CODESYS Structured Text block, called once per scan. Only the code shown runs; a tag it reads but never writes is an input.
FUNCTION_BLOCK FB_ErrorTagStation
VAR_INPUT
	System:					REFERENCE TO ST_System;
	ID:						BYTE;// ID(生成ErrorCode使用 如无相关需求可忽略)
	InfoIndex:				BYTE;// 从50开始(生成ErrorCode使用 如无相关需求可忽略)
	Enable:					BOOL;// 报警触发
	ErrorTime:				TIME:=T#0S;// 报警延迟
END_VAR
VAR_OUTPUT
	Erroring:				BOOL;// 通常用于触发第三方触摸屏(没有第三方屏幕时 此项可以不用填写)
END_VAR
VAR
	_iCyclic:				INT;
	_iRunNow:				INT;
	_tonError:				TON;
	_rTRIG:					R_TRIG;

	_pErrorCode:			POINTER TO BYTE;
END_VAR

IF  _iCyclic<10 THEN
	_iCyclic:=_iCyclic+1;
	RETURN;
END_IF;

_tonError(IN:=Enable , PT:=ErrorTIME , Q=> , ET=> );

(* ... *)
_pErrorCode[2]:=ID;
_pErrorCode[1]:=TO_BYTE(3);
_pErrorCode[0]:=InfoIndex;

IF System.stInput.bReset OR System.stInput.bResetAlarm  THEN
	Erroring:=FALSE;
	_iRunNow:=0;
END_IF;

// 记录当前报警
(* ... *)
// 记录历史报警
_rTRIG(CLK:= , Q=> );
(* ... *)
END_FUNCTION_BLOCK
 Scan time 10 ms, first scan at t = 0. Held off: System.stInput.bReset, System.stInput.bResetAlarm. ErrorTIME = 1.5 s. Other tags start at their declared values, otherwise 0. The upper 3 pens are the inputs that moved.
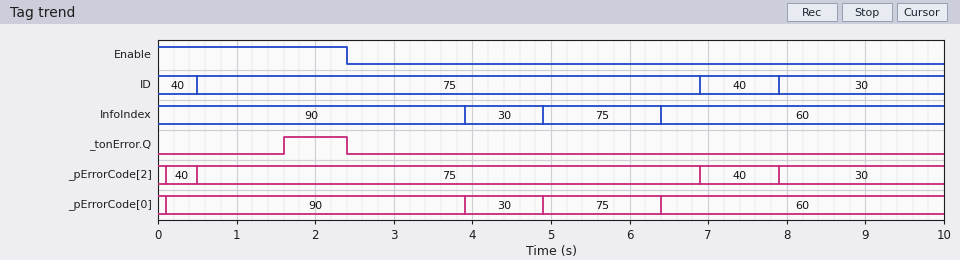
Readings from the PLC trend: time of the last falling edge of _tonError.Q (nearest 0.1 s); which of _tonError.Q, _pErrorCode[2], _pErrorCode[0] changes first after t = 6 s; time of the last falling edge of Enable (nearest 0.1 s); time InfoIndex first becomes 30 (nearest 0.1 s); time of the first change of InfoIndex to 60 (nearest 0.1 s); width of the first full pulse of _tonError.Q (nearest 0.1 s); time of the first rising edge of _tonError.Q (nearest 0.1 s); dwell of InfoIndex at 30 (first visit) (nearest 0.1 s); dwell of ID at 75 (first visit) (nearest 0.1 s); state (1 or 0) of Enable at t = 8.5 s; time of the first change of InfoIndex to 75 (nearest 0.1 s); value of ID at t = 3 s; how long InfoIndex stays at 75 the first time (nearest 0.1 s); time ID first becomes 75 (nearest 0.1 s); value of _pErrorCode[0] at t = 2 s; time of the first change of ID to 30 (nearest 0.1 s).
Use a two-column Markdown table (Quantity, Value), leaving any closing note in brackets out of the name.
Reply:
| Quantity | Value |
|---|---|
| time of the last falling edge of _tonError.Q | 2.4 s |
| which of _tonError.Q, _pErrorCode[2], _pErrorCode[0] changes first after t = 6 s | _pErrorCode[0] |
| time of the last falling edge of Enable | 2.4 s |
| time InfoIndex first becomes 30 | 3.9 s |
| time of the first change of InfoIndex to 60 | 6.4 s |
| width of the first full pulse of _tonError.Q | 0.8 s |
| time of the first rising edge of _tonError.Q | 1.6 s |
| dwell of InfoIndex at 30 (first visit) | 1.0 s |
| dwell of ID at 75 (first visit) | 6.4 s |
| state (1 or 0) of Enable at t = 8.5 s | 0 |
| time of the first change of InfoIndex to 75 | 4.9 s |
| value of ID at t = 3 s | 75 |
| how long InfoIndex stays at 75 the first time | 1.5 s |
| time ID first becomes 75 | 0.5 s |
| value of _pErrorCode[0] at t = 2 s | 90 |
| time of the first change of ID to 30 | 7.9 s |
